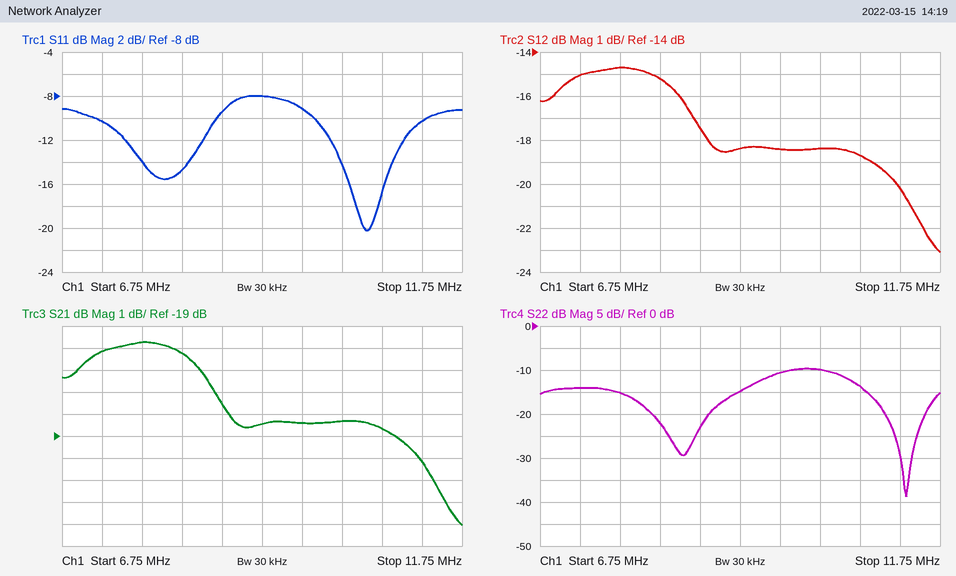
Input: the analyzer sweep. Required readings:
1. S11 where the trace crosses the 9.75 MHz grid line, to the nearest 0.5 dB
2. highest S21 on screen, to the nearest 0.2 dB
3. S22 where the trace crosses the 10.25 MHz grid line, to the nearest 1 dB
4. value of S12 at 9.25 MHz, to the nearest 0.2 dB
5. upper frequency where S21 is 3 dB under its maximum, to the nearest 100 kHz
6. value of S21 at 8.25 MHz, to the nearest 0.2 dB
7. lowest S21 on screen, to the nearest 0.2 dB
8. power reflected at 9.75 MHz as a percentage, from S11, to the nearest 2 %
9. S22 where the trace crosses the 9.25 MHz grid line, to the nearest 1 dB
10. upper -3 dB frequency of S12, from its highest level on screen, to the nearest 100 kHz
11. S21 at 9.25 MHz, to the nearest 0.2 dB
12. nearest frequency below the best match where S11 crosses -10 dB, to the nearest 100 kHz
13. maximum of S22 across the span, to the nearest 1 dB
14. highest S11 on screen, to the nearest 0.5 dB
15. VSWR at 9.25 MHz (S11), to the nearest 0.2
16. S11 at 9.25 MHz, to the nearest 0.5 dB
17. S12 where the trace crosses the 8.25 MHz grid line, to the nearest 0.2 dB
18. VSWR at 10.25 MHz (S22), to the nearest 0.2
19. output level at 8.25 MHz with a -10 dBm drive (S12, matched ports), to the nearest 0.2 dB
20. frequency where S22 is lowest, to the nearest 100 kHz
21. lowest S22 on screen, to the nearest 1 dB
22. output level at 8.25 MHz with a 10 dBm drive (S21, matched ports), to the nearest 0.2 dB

-9.0 dB
-14.8 dB
-10 dB
-18.4 dB
8.8 MHz
-15.2 dB
-23.0 dB
12 %
-15 dB
8.8 MHz
-18.4 dB
9.9 MHz
-10 dB
-8.0 dB
2.4
-8.0 dB
-15.2 dB
2.0
-25.2 dBm
11.3 MHz
-39 dB
-5.2 dBm
